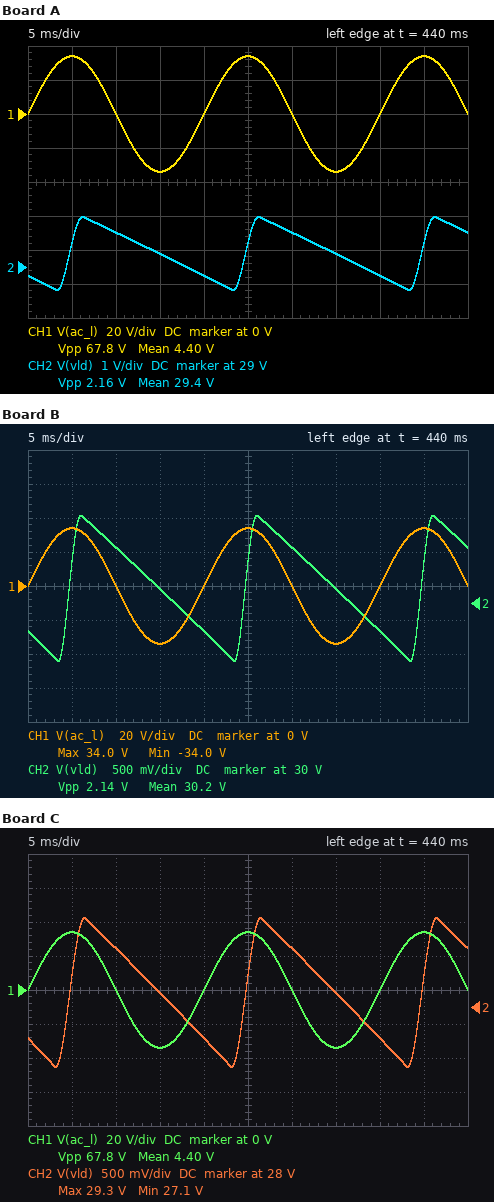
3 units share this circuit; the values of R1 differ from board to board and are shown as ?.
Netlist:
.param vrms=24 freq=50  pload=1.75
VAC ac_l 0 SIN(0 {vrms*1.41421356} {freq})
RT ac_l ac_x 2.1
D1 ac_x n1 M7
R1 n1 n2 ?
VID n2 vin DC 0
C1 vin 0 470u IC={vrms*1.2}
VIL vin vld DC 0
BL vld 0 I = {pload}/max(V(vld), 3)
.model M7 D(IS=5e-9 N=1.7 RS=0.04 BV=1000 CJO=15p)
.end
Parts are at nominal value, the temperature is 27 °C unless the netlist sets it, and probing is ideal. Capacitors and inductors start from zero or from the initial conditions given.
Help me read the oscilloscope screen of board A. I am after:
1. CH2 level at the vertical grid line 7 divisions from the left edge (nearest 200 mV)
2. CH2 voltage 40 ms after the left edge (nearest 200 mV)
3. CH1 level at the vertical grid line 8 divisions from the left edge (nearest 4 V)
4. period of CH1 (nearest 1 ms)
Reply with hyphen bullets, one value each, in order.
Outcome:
- 29.4 V
- 28.8 V
- 0 V
- 20 ms
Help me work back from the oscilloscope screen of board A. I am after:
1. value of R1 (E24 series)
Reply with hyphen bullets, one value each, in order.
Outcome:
- 3.9 Ω
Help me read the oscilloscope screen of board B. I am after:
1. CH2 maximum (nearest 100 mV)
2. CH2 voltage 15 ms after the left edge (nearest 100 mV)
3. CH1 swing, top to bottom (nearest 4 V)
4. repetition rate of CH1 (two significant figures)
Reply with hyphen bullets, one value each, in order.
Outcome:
- 31.3 V
- 30.2 V
- 68 V
- 50 Hz
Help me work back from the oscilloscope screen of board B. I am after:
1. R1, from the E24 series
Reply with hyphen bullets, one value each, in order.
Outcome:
- 2 Ω
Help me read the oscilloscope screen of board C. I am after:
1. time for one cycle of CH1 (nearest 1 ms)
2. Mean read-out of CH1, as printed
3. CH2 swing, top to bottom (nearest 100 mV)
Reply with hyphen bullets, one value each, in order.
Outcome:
- 20 ms
- 4.40 V
- 2.2 V
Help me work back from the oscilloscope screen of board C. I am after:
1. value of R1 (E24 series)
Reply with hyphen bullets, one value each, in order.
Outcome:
- 6.8 Ω
